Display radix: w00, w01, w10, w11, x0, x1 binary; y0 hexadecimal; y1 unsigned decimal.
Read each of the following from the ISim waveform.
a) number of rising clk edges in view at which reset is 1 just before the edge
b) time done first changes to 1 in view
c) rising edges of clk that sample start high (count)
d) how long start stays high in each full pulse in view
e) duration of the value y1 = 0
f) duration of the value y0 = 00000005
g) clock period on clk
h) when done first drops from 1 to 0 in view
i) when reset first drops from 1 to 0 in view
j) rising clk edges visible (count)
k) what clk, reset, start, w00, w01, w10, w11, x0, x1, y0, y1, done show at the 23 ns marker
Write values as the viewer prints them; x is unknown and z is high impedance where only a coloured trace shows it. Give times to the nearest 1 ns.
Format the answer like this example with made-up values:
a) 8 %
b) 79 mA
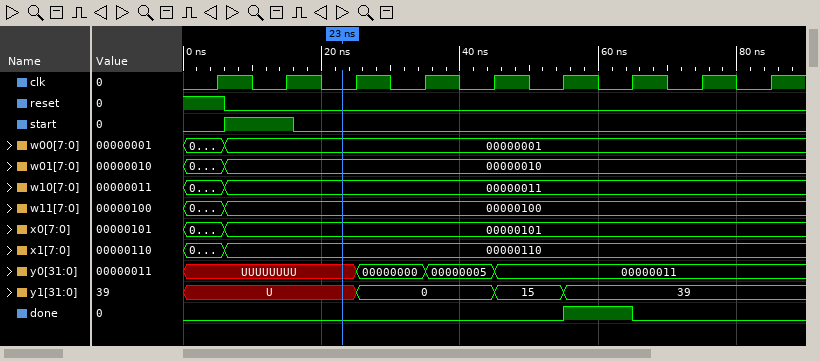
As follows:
a) 1
b) 55 ns
c) 1
d) 10 ns
e) 20 ns
f) 10 ns
g) 10 ns
h) 65 ns
i) 6 ns
j) 9
k) clk=0, reset=0, start=0, w00=00000001, w01=00000010, w10=00000011, w11=00000100, x0=00000101, x1=00000110, y0=UUUUUUUU, y1=U, done=0
